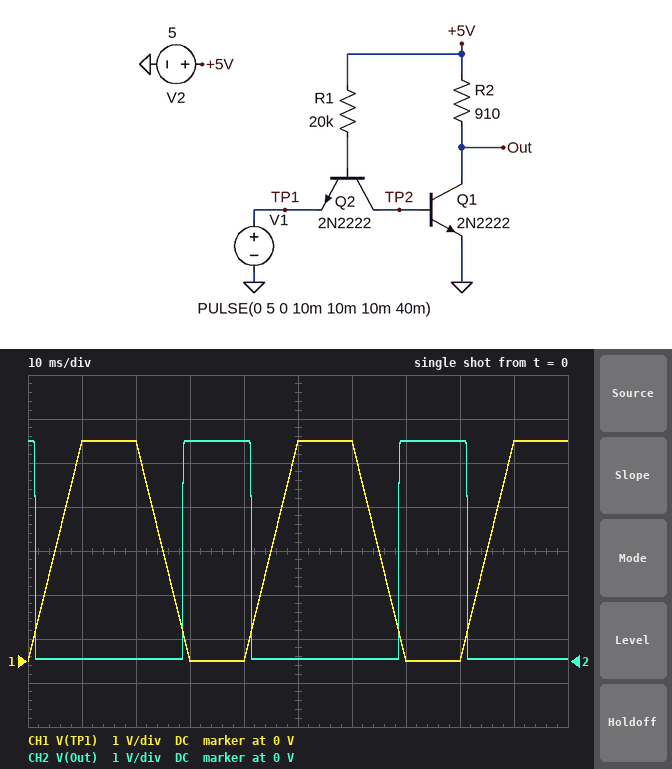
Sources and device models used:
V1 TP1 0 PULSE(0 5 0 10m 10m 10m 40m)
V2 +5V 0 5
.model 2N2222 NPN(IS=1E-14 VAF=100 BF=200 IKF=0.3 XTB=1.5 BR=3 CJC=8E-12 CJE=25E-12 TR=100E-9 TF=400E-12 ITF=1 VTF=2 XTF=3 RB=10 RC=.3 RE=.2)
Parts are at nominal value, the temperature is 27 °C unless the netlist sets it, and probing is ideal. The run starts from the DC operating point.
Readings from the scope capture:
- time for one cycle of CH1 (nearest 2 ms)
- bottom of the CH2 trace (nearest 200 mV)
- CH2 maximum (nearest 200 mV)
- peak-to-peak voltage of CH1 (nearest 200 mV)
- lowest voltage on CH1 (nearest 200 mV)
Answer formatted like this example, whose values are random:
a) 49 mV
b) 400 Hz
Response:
a) 40 ms
b) 0 V
c) 5.0 V
d) 5.0 V
e) 0 V
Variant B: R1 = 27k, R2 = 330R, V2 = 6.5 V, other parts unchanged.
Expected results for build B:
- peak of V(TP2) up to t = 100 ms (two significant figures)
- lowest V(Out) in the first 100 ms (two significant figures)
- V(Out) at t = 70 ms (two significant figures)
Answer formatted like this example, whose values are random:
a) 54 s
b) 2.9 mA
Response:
a) 750 mV
b) 75 mV
c) 6.5 V
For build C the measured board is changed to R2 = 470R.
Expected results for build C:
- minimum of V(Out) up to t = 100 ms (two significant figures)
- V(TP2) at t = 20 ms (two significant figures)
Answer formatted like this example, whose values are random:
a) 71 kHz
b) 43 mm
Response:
a) 56 mV
b) 730 mV
